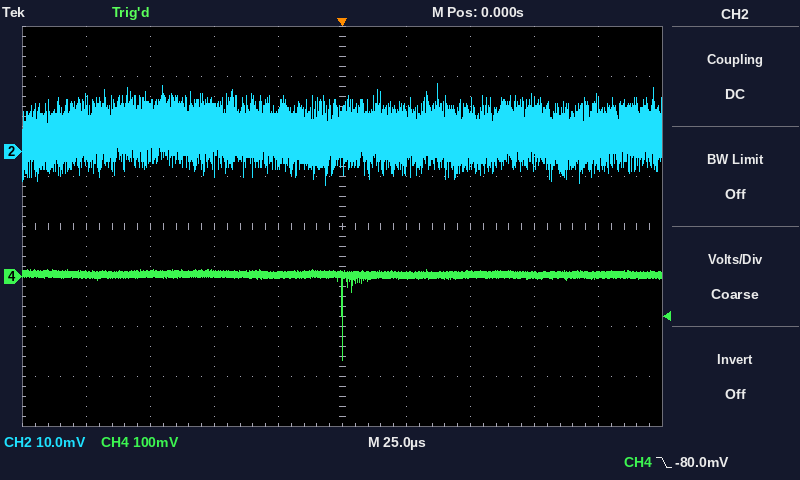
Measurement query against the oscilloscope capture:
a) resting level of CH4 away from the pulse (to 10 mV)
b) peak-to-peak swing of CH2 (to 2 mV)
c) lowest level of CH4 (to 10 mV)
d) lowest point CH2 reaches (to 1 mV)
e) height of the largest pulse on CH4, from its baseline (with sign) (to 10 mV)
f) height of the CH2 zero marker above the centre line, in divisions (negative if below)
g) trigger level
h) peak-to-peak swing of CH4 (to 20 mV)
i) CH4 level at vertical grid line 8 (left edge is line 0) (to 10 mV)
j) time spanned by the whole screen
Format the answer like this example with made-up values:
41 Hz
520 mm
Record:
0 mV
20 mV
-170 mV
-7 mV
-170 mV
+1.5 div
-80.0 mV
180 mV
0 mV
250 µs
